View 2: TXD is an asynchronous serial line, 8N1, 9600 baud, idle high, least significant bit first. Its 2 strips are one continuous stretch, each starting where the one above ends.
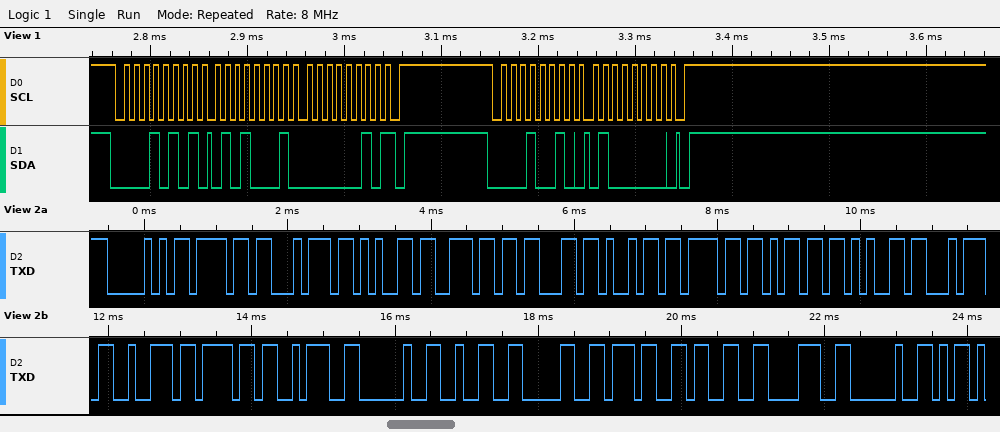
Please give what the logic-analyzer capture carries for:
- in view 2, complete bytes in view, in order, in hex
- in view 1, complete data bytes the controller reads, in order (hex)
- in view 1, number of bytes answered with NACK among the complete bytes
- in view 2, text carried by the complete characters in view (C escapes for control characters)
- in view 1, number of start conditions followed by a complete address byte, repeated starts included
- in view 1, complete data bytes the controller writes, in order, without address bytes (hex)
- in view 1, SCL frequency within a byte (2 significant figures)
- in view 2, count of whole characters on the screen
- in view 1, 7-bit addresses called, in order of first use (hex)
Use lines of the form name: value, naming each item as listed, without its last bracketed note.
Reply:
in view 2, complete bytes in view, in order, in hex: 50 6F 74 65 6E 63 69 6F 6D 65 74 72 6F 3A 20 32 30 37 33 38 20
in view 1, complete data bytes the controller reads, in order: 51 02
in view 1, number of bytes answered with NACK among the complete bytes: 1
in view 2, text carried by the complete characters in view: "Potenciometro: 20738 "
in view 1, number of start conditions followed by a complete address byte, repeated starts included: 2
in view 1, complete data bytes the controller writes, in order, without address bytes: 40
in view 1, SCL frequency within a byte: 100 kHz
in view 2, count of whole characters on the screen: 21
in view 1, 7-bit addresses called, in order of first use: 0x0A 0x09
